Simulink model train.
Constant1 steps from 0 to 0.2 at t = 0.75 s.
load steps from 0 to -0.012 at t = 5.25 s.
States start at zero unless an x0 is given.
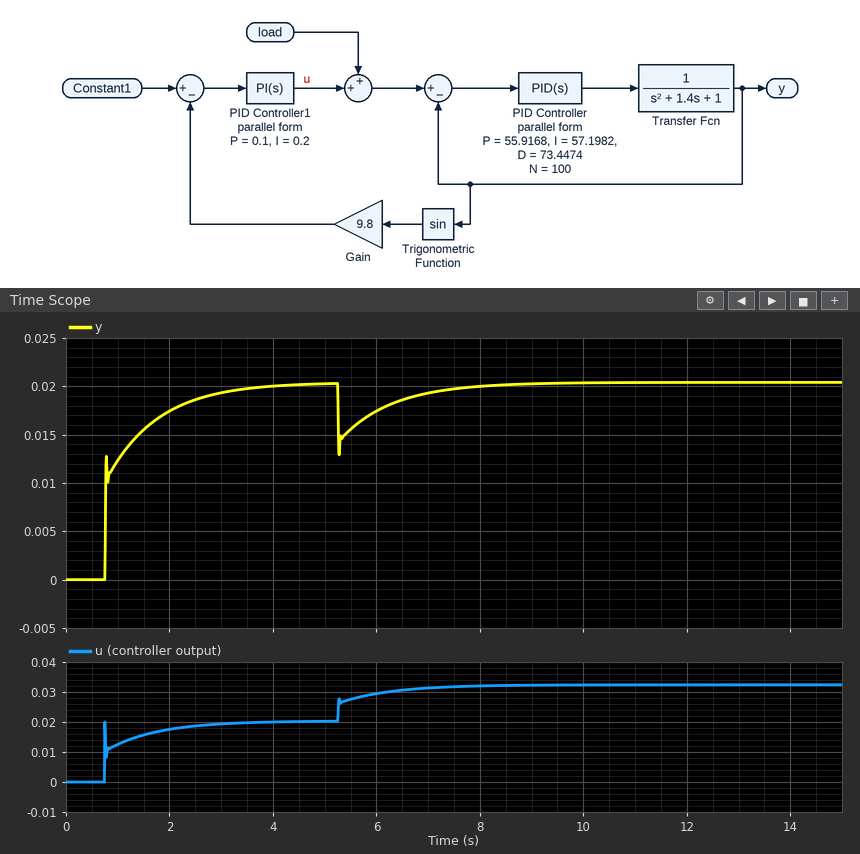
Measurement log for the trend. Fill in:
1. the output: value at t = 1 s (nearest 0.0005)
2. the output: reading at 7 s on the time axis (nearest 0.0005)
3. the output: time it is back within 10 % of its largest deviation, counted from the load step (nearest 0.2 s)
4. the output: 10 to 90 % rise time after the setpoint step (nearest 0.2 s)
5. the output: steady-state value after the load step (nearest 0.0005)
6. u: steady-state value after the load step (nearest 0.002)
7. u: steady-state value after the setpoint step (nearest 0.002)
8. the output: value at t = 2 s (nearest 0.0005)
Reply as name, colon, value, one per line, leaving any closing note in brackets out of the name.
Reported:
the output: value at t = 1 s: 0.0125
the output: reading at 7 s on the time axis: 0.0195
the output: time it is back within 10 % of its largest deviation, counted from the load step: 2.2 s
the output: 10 to 90 % rise time after the setpoint step: 1.6 s
the output: steady-state value after the load step: 0.0205
u: steady-state value after the load step: 0.032
u: steady-state value after the setpoint step: 0.020
the output: value at t = 2 s: 0.0175
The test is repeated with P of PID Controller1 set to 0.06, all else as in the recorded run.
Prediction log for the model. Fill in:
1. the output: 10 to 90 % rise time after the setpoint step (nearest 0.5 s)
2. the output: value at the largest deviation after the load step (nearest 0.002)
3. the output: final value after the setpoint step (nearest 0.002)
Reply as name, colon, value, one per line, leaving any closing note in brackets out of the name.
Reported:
the output: 10 to 90 % rise time after the setpoint step: 1.5 s
the output: value at the largest deviation after the load step: 0.012
the output: final value after the setpoint step: 0.020
